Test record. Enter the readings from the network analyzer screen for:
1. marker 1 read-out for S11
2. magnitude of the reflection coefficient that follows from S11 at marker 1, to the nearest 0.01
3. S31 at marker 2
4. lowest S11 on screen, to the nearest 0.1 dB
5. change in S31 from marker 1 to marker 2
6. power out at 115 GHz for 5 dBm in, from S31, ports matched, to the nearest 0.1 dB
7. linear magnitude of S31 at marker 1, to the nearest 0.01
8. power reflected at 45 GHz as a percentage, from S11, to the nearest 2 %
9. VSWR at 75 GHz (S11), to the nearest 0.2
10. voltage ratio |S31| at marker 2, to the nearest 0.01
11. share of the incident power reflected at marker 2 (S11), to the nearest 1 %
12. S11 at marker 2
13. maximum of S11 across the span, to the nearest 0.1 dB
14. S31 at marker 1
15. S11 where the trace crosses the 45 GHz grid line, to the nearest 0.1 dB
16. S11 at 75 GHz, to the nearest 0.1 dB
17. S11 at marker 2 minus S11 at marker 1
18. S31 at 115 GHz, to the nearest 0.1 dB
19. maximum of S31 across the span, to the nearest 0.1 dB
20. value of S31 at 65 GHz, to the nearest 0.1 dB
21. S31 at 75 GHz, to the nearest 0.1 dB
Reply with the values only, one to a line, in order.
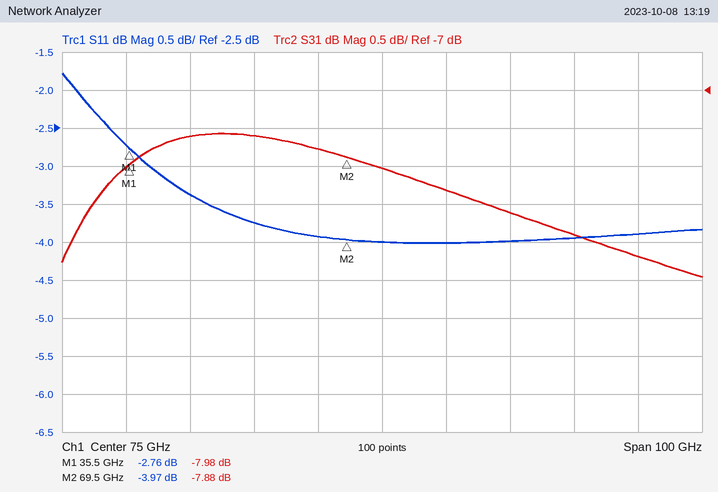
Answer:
-2.76 dB
0.73
-7.88 dB
-4.0 dB
0.10 dB
-4.2 dBm
0.40
46 %
4.4
0.40
40 %
-3.97 dB
-1.8 dB
-7.98 dB
-3.4 dB
-4.0 dB
-1.21 dB
-9.2 dB
-7.6 dB
-7.8 dB
-8.0 dB
